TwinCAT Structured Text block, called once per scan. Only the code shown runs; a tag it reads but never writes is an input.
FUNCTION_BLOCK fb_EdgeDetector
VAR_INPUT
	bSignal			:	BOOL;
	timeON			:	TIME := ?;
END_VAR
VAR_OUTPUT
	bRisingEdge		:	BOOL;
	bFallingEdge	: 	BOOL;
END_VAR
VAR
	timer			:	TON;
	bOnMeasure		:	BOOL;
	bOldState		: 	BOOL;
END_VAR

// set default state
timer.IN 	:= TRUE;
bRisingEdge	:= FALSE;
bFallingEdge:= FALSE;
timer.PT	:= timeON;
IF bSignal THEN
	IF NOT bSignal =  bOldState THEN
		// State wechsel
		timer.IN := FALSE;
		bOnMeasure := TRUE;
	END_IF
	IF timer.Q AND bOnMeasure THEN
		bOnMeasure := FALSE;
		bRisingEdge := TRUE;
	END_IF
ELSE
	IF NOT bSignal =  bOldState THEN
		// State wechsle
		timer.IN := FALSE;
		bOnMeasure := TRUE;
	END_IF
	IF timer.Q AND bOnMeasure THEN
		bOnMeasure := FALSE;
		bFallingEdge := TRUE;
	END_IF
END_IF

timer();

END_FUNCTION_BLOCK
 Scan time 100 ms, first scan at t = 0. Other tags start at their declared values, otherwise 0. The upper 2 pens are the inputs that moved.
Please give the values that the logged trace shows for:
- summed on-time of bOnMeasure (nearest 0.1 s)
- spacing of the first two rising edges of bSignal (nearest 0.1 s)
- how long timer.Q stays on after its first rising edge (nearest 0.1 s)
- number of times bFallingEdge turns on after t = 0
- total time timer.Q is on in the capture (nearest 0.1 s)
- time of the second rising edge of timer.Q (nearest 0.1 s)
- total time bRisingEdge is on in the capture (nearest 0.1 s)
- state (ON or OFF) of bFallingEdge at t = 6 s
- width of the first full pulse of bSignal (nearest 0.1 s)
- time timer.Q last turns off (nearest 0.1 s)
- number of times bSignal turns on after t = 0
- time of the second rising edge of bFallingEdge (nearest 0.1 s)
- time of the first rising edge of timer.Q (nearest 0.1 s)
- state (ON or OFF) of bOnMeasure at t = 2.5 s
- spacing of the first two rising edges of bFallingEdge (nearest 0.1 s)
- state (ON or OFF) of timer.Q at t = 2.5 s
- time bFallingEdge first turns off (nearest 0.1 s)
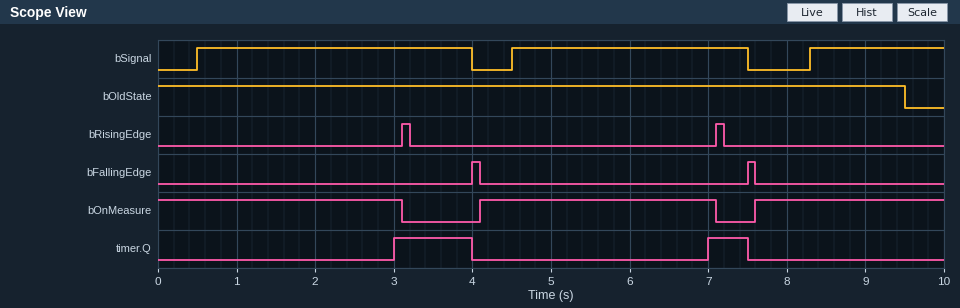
8.5 s
4.0 s
1.0 s
2
1.5 s
7.0 s
0.2 s
OFF
3.5 s
7.5 s
3
7.5 s
3.0 s
ON
3.5 s
OFF
4.1 s
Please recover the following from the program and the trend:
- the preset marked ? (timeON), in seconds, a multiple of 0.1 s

2.5 s
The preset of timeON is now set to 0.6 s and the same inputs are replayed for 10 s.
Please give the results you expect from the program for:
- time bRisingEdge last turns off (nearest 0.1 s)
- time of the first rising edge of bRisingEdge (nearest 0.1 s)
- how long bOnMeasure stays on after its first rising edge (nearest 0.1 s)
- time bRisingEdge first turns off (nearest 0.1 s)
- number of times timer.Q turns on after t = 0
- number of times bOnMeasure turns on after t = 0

9.6 s
1.2 s
1.1 s
1.3 s
3
3
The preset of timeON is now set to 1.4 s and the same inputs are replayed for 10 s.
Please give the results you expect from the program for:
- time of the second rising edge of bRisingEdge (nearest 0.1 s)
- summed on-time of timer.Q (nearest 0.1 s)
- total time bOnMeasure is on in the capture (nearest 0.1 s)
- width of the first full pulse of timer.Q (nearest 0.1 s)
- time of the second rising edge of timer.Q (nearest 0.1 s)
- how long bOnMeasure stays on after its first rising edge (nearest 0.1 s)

6.0 s
3.7 s
6.3 s
2.1 s
5.9 s
1.9 s
